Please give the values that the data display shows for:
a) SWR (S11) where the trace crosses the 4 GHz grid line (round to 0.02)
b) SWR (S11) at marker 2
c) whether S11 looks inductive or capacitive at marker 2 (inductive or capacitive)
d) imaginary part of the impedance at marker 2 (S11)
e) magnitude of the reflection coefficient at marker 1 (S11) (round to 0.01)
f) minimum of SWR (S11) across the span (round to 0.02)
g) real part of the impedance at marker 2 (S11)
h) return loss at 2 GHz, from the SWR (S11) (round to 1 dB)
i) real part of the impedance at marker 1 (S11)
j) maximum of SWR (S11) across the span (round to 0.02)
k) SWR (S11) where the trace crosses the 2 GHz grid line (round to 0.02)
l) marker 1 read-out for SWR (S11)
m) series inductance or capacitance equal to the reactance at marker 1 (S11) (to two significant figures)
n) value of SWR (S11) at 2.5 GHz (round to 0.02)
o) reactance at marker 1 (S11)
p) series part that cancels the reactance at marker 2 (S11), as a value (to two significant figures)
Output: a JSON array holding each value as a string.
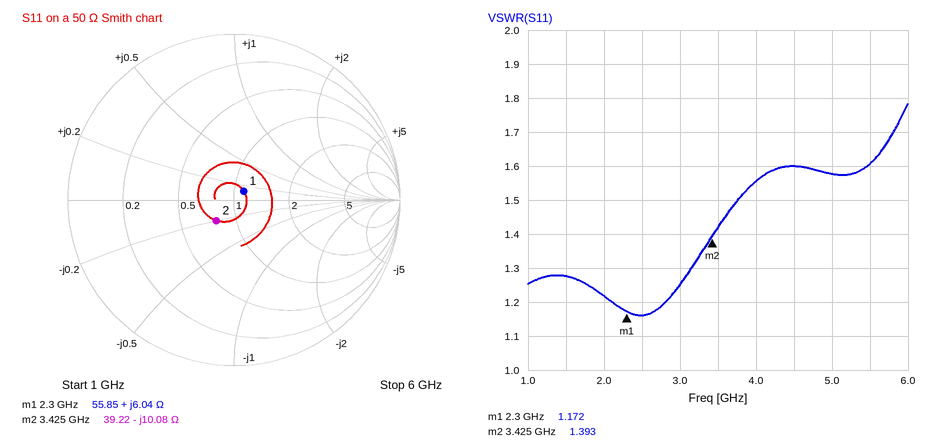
["1.56", "1.393", "capacitive", "-10.08 Ω", "0.08", "1.16", "39.22 Ω", "20 dB", "55.85 Ω", "1.78", "1.22", "1.172", "420 pH", "1.16", "+6.04 Ω", "470 pH"]
